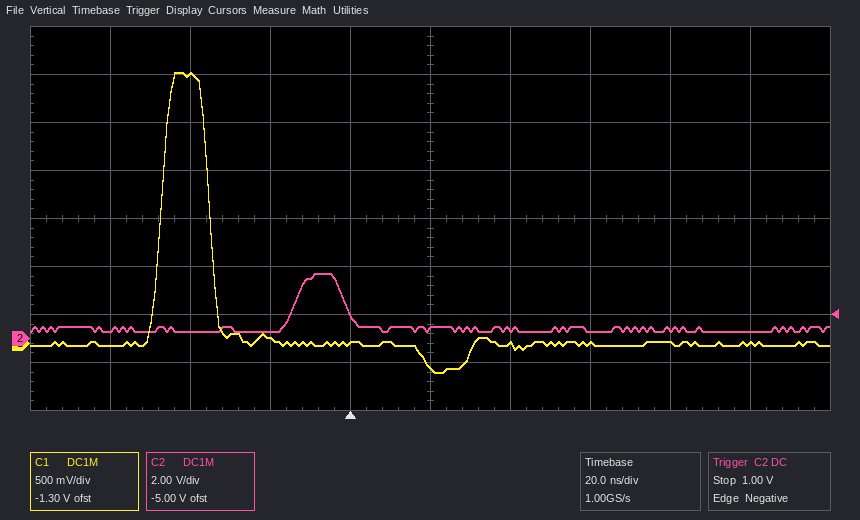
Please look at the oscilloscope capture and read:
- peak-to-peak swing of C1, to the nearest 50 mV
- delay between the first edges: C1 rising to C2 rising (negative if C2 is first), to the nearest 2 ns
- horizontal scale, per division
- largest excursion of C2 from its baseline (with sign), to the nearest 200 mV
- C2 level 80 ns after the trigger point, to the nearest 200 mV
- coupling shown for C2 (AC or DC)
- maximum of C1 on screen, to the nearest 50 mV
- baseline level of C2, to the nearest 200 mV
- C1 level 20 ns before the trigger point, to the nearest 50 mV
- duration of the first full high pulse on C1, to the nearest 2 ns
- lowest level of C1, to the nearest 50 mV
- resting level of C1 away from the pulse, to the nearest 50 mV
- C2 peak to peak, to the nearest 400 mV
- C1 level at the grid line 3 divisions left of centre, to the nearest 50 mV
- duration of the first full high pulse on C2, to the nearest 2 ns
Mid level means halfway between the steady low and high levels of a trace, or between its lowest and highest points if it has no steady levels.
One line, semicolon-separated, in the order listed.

3.10 V; +34 ns; 20 ns; +2.4 V; 400 mV; DC; 2.80 V; 400 mV; 50 mV; 12 ns; -300 mV; 0 mV; 2.4 V; 2.80 V; 12 ns
